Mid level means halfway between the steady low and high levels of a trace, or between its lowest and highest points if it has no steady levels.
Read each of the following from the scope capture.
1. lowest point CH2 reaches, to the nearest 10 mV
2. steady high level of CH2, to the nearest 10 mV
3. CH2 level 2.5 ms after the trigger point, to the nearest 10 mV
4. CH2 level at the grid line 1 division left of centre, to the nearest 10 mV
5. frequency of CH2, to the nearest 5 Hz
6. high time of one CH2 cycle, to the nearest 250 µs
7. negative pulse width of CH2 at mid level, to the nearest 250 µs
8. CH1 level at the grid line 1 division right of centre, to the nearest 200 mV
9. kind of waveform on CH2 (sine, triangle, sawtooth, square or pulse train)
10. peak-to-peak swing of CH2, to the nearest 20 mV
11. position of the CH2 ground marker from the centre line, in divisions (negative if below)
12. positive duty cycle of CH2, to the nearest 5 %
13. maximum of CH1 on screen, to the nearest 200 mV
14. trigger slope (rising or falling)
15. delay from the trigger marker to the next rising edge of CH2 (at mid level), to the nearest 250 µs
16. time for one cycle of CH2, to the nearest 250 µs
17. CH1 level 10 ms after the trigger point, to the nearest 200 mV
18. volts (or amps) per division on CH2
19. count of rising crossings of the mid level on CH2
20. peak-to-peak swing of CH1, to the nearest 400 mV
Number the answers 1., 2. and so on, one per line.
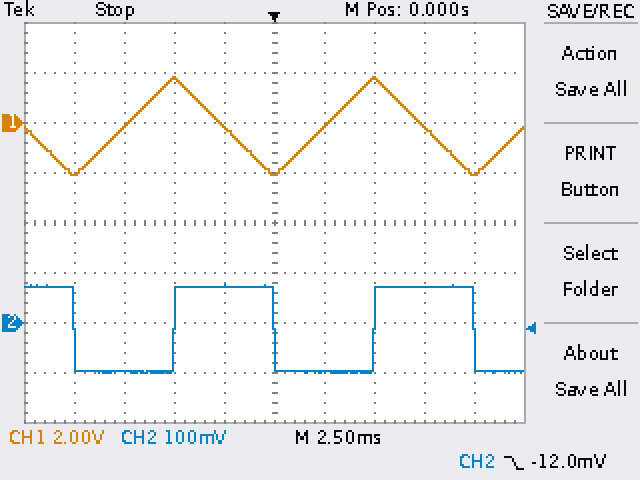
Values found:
1. -100 mV
2. 70 mV
3. -100 mV
4. 70 mV
5. 100 Hz
6. 5.00 ms
7. 5.00 ms
8. -200 mV
9. square
10. 180 mV
11. -2.0 div
12. 50 %
13. 1.8 V
14. falling
15. 5.00 ms
16. 10.00 ms
17. -2.0 V
18. 100 mV
19. 2
20. 4.0 V
